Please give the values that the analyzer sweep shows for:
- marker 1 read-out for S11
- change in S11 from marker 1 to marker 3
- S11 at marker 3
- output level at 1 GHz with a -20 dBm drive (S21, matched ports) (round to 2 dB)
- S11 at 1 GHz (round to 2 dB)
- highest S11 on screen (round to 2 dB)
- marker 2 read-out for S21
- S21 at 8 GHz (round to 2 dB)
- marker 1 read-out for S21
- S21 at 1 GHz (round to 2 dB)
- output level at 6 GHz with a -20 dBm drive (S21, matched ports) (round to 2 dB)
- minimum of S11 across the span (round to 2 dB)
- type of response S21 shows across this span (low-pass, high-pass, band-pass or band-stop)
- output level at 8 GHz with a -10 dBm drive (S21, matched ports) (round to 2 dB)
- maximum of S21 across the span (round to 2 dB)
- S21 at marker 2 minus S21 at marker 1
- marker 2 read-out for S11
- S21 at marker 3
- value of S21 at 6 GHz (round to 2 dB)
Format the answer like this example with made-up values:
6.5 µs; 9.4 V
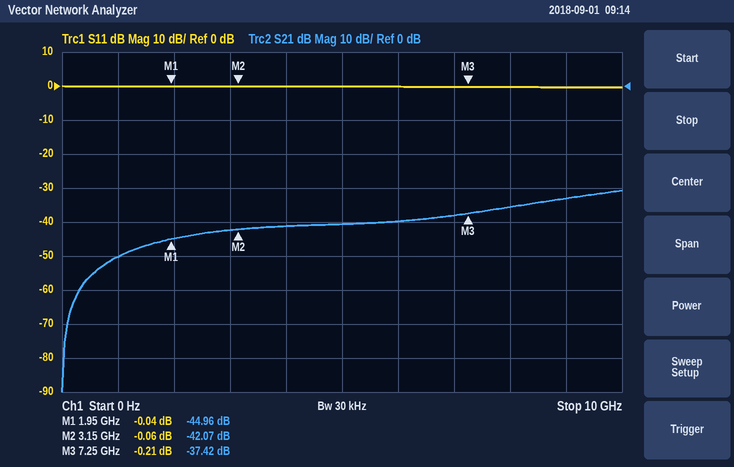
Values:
-0.04 dB; -0.17 dB; -0.21 dB; -70 dBm; 0 dB; 0 dB; -42.07 dB; -36 dB; -44.96 dB; -50 dB; -60 dBm; 0 dB; high-pass; -46 dBm; -30 dB; 2.89 dB; -0.06 dB; -37.42 dB; -40 dB
